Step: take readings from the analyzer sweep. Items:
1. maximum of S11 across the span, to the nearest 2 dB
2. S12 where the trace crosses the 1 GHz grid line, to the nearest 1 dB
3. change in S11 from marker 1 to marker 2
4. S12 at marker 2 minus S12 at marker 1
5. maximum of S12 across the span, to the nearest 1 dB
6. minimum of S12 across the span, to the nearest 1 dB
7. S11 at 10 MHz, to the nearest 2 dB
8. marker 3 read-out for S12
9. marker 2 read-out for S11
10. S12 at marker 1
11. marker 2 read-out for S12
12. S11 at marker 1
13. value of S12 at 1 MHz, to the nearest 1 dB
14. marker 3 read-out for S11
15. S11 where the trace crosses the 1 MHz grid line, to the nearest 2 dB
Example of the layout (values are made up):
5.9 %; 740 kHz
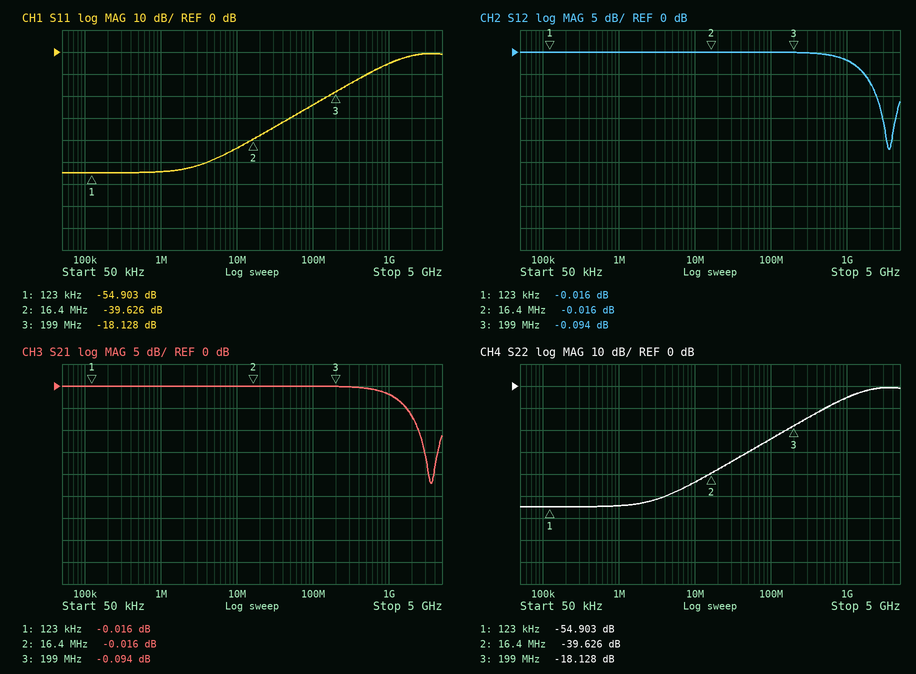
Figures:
0 dB; -2 dB; 15.277 dB; 0.000 dB; 0 dB; -22 dB; -44 dB; -0.094 dB; -39.626 dB; -0.016 dB; -0.016 dB; -54.903 dB; 0 dB; -18.128 dB; -54 dB
